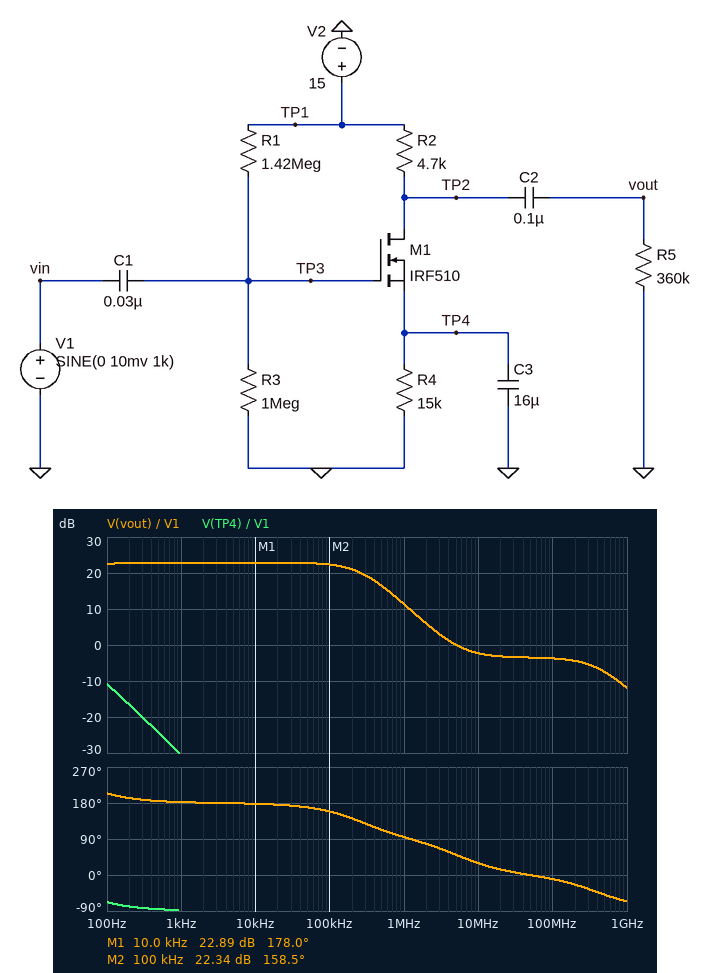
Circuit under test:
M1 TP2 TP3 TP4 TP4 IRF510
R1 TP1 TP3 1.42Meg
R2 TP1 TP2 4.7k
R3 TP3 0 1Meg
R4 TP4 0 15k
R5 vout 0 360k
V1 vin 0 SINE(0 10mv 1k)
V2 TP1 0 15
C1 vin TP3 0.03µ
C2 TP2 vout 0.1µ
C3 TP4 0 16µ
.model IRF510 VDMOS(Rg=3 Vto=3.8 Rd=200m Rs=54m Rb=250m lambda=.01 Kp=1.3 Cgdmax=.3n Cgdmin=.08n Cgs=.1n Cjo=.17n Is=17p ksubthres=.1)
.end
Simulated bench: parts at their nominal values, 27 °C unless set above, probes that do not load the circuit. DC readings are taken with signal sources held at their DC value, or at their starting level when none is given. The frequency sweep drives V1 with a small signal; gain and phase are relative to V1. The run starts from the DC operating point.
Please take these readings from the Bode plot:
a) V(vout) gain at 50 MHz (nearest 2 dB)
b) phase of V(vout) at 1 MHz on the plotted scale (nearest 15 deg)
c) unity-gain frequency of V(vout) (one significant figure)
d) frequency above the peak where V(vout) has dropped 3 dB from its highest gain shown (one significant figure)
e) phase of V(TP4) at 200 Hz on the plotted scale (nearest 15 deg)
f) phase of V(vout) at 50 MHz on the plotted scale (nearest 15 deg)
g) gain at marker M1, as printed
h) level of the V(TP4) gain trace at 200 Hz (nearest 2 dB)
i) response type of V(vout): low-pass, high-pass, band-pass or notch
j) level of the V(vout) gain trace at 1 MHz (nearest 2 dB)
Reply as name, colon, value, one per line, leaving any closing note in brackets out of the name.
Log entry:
V(vout) gain at 50 MHz: -4 dB
phase of V(vout) at 1 MHz on the plotted scale: 90 deg
unity-gain frequency of V(vout): 5 MHz
frequency above the peak where V(vout) has dropped 3 dB from its highest gain shown: 300 kHz
phase of V(TP4) at 200 Hz on the plotted scale: -75 deg
phase of V(vout) at 50 MHz on the plotted scale: 0 deg
gain at marker M1, as printed: 22.89 dB
level of the V(TP4) gain trace at 200 Hz: -16 dB
response type of V(vout): low-pass, high-pass, band-pass or notch: low-pass
level of the V(vout) gain trace at 1 MHz: 12 dB
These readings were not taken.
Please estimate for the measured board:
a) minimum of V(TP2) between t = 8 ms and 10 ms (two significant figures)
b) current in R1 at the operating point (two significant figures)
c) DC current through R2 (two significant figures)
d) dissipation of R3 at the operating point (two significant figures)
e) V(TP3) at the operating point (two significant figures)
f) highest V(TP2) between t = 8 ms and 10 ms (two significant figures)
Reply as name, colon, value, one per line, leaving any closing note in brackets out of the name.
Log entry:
minimum of V(TP2) between t = 8 ms and 10 ms: 14 V
current in R1 at the operating point: 6.2 µA
DC current through R2: 170 µA
dissipation of R3 at the operating point: 38 µW
V(TP3) at the operating point: 6.2 V
highest V(TP2) between t = 8 ms and 10 ms: 14 V
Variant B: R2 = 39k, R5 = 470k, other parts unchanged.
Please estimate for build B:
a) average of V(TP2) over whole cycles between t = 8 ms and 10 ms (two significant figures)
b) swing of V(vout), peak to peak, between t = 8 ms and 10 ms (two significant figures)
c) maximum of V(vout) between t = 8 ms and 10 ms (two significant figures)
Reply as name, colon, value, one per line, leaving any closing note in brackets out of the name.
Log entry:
average of V(TP2) over whole cycles between t = 8 ms and 10 ms: 8.3 V
swing of V(vout), peak to peak, between t = 8 ms and 10 ms: 1.5 V
maximum of V(vout) between t = 8 ms and 10 ms: 740 mV
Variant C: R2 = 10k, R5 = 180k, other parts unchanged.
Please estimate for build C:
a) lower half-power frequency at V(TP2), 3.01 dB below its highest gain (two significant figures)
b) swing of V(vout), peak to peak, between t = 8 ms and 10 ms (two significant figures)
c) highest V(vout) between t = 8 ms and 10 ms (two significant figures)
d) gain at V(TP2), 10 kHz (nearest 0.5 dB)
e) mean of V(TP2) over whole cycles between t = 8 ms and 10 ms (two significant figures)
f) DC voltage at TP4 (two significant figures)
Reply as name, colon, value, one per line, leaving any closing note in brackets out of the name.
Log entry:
lower half-power frequency at V(TP2), 3.01 dB below its highest gain: 31 Hz
swing of V(vout), peak to peak, between t = 8 ms and 10 ms: 540 mV
highest V(vout) between t = 8 ms and 10 ms: 260 mV
gain at V(TP2), 10 kHz: 28.5 dB
mean of V(TP2) over whole cycles between t = 8 ms and 10 ms: 13 V
DC voltage at TP4: 2.6 V
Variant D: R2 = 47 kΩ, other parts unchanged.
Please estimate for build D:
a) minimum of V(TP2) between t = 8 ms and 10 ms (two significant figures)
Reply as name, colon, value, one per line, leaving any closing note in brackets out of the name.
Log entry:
minimum of V(TP2) between t = 8 ms and 10 ms: 6.2 V
